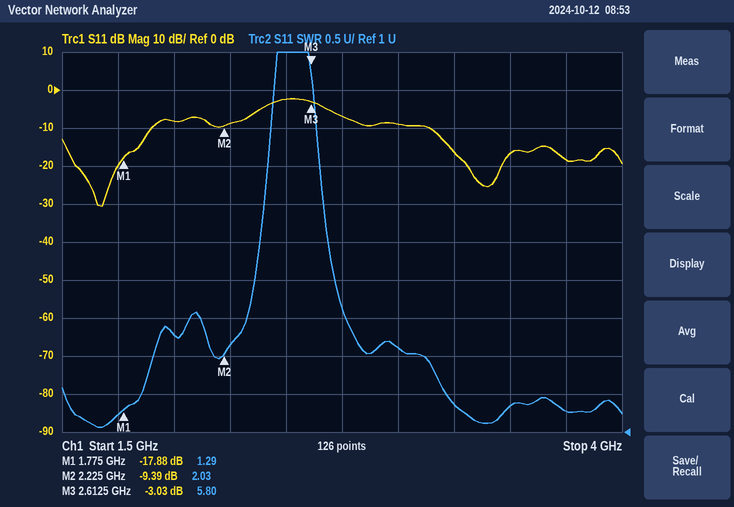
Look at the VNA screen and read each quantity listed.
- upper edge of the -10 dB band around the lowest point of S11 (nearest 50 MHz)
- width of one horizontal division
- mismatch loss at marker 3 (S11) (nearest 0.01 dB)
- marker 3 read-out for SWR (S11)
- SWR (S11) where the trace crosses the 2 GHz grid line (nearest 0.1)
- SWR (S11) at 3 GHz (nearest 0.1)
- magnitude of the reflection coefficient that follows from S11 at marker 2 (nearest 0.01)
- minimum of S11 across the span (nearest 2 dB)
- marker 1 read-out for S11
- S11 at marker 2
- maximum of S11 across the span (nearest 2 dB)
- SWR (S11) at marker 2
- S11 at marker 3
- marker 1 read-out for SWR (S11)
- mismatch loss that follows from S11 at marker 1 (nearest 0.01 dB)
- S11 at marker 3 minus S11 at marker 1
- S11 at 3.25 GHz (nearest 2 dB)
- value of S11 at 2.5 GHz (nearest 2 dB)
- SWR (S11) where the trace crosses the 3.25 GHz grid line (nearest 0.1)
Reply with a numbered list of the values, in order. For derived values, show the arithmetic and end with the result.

1. 1.90 GHz
2. 250 MHz
3. −10 log10(1 − 10^(-3.03/10)) ≈ 2.99 dB
4. 5.80
5. 2.3
6. 2.1
7. 10^(-9.39/20) ≈ 0.34
8. -30 dB
9. -17.88 dB
10. -9.39 dB
11. -2 dB
12. 2.03
13. -3.03 dB
14. 1.29
15. −10 log10(1 − 10^(-17.88/10)) ≈ 0.07 dB
16. -3.03 − (-17.88) = 14.85 dB
17. -16 dB
18. -2 dB
19. 1.4
